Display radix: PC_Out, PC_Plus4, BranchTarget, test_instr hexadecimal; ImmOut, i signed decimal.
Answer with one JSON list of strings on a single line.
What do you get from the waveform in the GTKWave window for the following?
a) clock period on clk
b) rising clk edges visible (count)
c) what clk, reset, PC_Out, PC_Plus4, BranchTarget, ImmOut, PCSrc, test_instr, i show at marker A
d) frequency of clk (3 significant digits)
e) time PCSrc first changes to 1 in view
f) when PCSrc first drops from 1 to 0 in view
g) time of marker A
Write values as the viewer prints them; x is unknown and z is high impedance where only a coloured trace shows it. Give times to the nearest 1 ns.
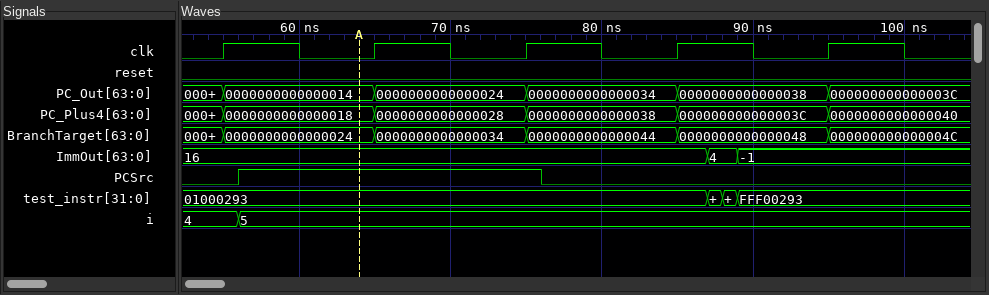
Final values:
["10 ns", "5", "clk=0, reset=0, PC_Out=0000000000000014, PC_Plus4=0000000000000018, BranchTarget=0000000000000024, ImmOut=16, PCSrc=1, test_instr=01000293, i=5", "100 MHz", "56 ns", "76 ns", "64 ns"]
